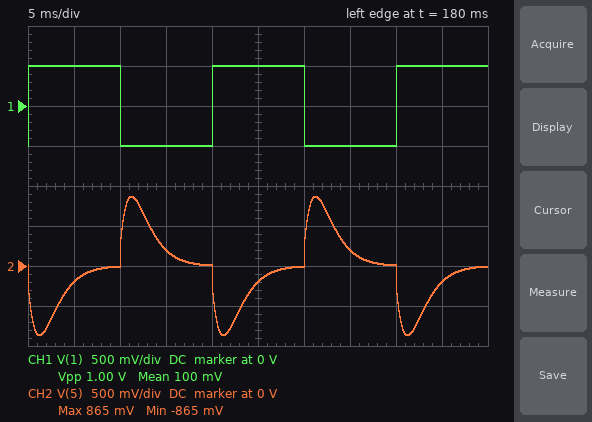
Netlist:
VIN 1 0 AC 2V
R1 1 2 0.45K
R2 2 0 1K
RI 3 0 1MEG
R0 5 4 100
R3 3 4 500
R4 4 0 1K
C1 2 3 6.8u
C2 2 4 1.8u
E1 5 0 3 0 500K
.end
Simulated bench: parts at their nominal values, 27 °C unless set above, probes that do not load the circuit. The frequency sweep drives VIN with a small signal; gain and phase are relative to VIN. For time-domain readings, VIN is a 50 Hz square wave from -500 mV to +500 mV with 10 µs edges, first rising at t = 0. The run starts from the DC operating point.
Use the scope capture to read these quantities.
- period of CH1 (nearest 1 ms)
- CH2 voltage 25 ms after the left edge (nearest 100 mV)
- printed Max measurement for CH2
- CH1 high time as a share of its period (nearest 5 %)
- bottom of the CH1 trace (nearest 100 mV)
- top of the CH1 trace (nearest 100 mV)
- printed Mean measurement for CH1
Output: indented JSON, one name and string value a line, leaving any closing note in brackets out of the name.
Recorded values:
{
  "period of CH1": "20 ms",
  "CH2 voltage 25 ms after the left edge": "-200 mV",
  "printed Max measurement for CH2": "865 mV",
  "CH1 high time as a share of its period": "50 %",
  "bottom of the CH1 trace": "-500 mV",
  "top of the CH1 trace": "500 mV",
  "printed Mean measurement for CH1": "100 mV"
}
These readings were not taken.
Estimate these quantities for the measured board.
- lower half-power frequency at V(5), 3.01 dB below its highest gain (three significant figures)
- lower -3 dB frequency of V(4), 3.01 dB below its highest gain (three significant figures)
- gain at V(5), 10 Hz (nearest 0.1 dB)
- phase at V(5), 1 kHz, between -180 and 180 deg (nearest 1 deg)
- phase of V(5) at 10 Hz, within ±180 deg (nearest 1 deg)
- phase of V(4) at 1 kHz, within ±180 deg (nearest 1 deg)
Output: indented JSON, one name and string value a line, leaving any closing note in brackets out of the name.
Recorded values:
{
  "lower half-power frequency at V(5), 3.01 dB below its highest gain": "49.2 Hz",
  "lower -3 dB frequency of V(4), 3.01 dB below its highest gain": "48.9 Hz",
  "gain at V(5), 10 Hz": "-14.1 dB",
  "phase at V(5), 1 kHz, between -180 and 180 deg": "143 deg",
  "phase of V(5) at 10 Hz, within ±180 deg": "-99 deg",
  "phase of V(4) at 1 kHz, within ±180 deg": "103 deg"
}
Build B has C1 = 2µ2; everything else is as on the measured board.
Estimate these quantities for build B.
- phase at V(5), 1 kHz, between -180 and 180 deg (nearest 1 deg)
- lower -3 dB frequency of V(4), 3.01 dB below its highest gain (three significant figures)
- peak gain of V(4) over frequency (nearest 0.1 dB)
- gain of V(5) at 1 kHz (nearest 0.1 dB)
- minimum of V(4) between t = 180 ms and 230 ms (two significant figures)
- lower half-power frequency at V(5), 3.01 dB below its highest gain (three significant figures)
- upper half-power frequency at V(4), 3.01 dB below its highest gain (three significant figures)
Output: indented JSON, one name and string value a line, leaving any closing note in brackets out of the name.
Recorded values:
{
  "phase at V(5), 1 kHz, between -180 and 180 deg": "146 deg",
  "lower -3 dB frequency of V(4), 3.01 dB below its highest gain": "98.2 Hz",
  "peak gain of V(4) over frequency": "-4.3 dB",
  "gain of V(5) at 1 kHz": "-8.9 dB",
  "minimum of V(4) between t = 180 ms and 230 ms": "-410 mV",
  "lower half-power frequency at V(5), 3.01 dB below its highest gain": "99.4 Hz",
  "upper half-power frequency at V(4), 3.01 dB below its highest gain": "420 Hz"
}
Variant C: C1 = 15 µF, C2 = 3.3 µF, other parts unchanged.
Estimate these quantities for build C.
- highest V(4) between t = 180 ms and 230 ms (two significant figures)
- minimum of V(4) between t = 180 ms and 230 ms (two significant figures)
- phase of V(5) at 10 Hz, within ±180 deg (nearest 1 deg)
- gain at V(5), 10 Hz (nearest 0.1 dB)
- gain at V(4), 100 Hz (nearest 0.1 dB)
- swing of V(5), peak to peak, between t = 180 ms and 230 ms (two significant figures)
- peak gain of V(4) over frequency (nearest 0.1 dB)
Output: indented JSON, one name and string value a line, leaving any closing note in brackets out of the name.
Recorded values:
{
  "highest V(4) between t = 180 ms and 230 ms": "590 mV",
  "minimum of V(4) between t = 180 ms and 230 ms": "-590 mV",
  "phase of V(5) at 10 Hz, within ±180 deg": "-109 deg",
  "gain at V(5), 10 Hz": "-7.5 dB",
  "gain at V(4), 100 Hz": "-2.0 dB",
  "swing of V(5), peak to peak, between t = 180 ms and 230 ms": "1.6 V",
  "peak gain of V(4) over frequency": "-0.8 dB"
}
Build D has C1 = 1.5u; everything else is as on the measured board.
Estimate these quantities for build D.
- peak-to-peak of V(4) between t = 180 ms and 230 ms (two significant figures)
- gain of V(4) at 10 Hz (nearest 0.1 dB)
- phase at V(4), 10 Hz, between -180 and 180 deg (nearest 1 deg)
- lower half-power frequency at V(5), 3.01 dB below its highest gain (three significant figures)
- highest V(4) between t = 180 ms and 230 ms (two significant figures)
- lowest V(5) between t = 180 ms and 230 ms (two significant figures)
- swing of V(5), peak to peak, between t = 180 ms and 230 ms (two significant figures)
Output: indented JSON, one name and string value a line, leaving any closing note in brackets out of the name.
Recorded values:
{
  "peak-to-peak of V(4) between t = 180 ms and 230 ms": "680 mV",
  "gain of V(4) at 10 Hz": "-29.8 dB",
  "phase at V(4), 10 Hz, between -180 and 180 deg": "-94 deg",
  "lower half-power frequency at V(5), 3.01 dB below its highest gain": "121 Hz",
  "highest V(4) between t = 180 ms and 230 ms": "340 mV",
  "lowest V(5) between t = 180 ms and 230 ms": "-540 mV",
  "swing of V(5), peak to peak, between t = 180 ms and 230 ms": "1.1 V"
}
